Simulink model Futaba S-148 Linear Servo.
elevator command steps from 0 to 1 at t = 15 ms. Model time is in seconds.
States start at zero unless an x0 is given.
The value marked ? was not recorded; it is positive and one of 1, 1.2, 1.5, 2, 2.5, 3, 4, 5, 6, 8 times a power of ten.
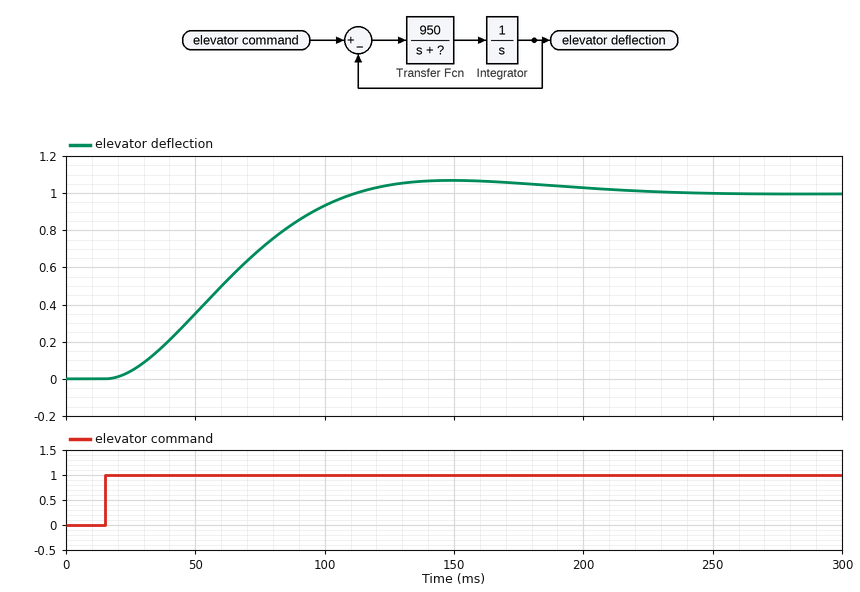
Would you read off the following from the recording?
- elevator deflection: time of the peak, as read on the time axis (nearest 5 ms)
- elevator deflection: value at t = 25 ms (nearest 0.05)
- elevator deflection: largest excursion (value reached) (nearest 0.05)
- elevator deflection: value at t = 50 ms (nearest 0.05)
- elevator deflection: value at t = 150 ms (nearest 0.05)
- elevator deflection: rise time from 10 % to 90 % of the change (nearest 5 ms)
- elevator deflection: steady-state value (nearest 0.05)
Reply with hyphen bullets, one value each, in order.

- 150 ms
- 0.05
- 1.05
- 0.35
- 1.05
- 65 ms
- 1.00
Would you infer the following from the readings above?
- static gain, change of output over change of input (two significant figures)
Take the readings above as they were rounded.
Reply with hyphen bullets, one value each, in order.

- 1.0
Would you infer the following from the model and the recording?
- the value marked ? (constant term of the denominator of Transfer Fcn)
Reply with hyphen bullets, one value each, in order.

- 40
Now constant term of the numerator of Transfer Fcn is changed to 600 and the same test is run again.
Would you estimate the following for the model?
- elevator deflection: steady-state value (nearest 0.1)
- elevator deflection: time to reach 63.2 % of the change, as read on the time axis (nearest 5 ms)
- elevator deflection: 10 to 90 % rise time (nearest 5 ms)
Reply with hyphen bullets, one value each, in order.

- 1.0
- 90 ms
- 105 ms
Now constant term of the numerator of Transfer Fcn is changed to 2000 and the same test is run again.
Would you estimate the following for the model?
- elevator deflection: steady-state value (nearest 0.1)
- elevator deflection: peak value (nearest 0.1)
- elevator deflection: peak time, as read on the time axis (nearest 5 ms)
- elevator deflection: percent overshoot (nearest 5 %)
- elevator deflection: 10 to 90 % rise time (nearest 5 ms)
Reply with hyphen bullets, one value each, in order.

- 1.0
- 1.2
- 95 ms
- 20 %
- 35 ms
